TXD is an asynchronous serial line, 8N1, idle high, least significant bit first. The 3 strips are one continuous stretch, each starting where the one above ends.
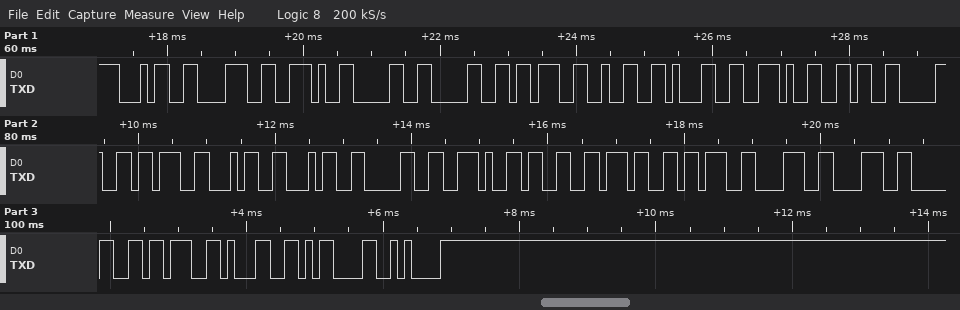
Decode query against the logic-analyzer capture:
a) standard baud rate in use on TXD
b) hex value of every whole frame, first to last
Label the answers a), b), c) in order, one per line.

a) 9600 baud
b) 34 38 2E 30 30 3B 32 31 2E 36 30 3B 34 34 30 2E 33 37 3B 38 38 30 3B 31 0D 0A
